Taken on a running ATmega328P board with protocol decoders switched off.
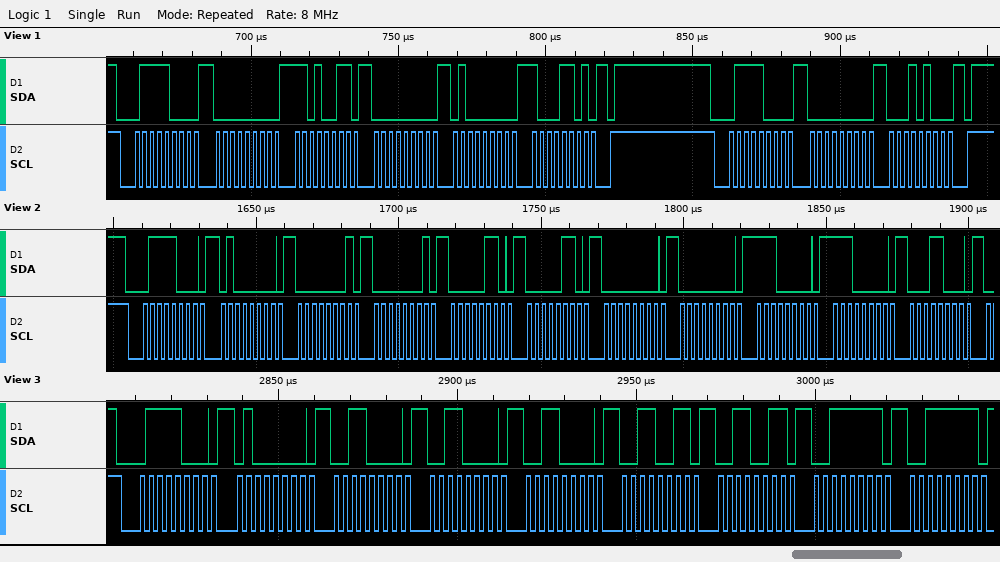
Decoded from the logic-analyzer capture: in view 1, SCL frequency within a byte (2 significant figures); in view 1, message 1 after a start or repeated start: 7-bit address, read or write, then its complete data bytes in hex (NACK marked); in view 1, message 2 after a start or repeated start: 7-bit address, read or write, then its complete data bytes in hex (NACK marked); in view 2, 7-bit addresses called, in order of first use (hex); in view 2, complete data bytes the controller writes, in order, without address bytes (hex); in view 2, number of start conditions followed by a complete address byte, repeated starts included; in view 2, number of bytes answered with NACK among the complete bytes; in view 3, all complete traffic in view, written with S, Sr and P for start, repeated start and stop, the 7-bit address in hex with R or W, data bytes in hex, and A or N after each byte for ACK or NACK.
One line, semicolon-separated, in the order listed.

400 kHz; 0x3C write: 00 D3 00 40 8D; 0x3C write: 00 14; 0x3C; 40 01 01 06 06 00 00 E0 E0 18; 1; 0; S 3CW A 40 A 30 A 30 A 30 A 33 A 33 A 3F A 3F A
